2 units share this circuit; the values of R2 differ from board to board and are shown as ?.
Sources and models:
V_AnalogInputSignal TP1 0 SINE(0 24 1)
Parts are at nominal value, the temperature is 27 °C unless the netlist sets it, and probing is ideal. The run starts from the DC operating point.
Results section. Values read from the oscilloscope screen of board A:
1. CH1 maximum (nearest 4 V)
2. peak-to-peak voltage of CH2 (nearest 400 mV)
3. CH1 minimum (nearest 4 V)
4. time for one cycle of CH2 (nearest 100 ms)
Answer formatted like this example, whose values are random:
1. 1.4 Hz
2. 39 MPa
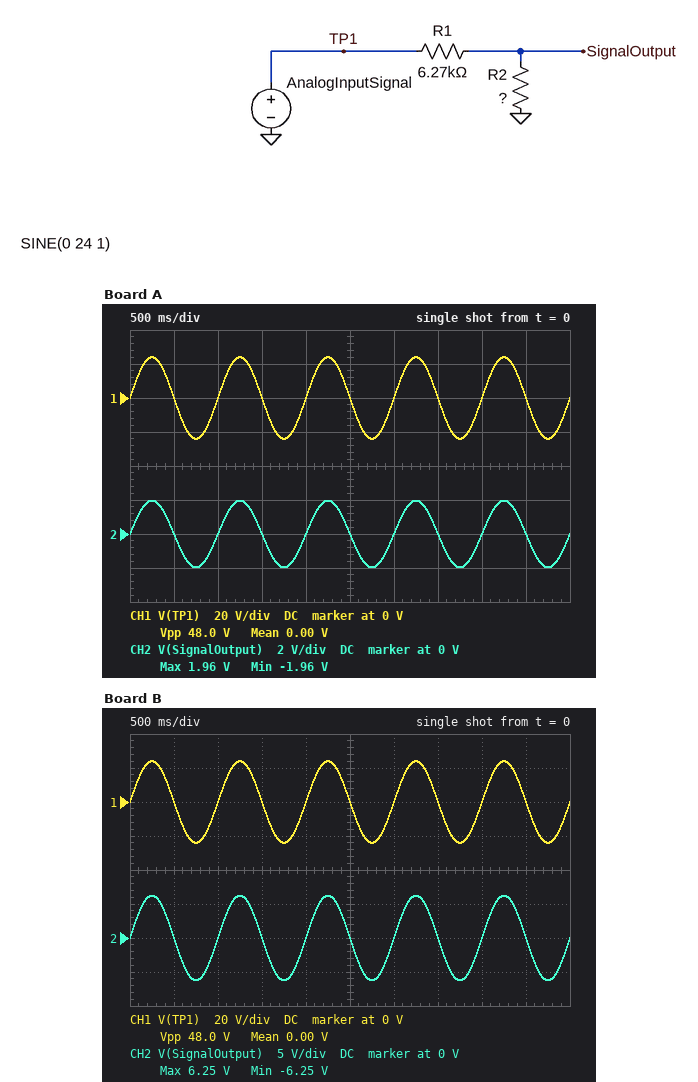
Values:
1. 24 V
2. 4.0 V
3. -24 V
4. 1.0 s
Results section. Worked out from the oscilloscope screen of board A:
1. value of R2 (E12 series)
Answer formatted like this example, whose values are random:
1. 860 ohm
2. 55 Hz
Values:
1. 560 Ω
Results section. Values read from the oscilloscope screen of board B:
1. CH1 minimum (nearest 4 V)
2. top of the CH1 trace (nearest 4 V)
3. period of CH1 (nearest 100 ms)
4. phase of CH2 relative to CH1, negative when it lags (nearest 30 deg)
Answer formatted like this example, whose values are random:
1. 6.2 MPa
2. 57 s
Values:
1. -24 V
2. 24 V
3. 1.0 s
4. 0 deg
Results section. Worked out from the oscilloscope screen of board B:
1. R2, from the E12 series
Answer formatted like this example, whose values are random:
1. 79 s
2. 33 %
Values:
1. 2.2 kΩ
